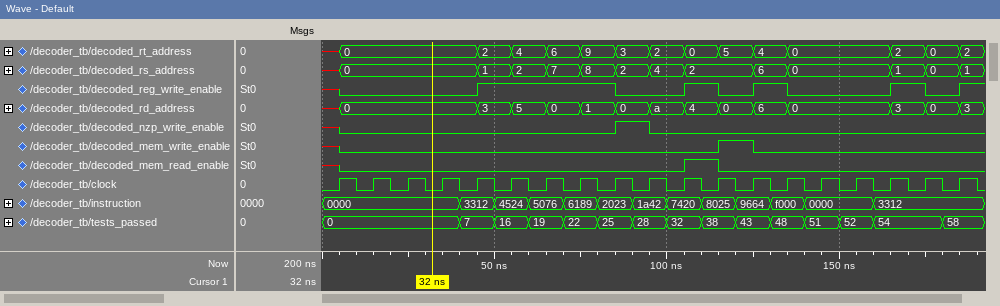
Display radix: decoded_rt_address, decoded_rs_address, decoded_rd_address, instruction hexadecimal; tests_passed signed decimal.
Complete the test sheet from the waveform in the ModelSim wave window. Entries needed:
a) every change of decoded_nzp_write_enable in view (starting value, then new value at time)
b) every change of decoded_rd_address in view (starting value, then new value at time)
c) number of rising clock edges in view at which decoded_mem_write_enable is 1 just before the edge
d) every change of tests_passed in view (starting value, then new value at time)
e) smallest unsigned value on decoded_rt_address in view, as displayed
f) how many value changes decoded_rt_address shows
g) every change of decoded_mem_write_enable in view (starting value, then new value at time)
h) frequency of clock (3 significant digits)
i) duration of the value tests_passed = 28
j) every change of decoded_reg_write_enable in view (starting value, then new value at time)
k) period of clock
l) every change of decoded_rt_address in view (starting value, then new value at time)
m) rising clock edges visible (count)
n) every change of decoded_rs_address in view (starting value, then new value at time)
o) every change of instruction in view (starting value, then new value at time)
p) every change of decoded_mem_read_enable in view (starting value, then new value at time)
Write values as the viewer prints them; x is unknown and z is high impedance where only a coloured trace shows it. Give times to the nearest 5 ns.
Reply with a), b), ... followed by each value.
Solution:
a) x, 0 at 5 ns, 1 at 85 ns, 0 at 95 ns
b) x, 0 at 5 ns, 3 at 45 ns, 5 at 55 ns, 0 at 65 ns, 1 at 75 ns, 0 at 85 ns, a at 95 ns, 4 at 105 ns, 0 at 115 ns, 6 at 125 ns, 0 at 135 ns, 3 at 165 ns, 0 at 175 ns, 3 at 185 ns
c) 1
d) 0, 7 at 40 ns, 16 at 50 ns, 19 at 60 ns, 22 at 70 ns, 25 at 80 ns, 28 at 90 ns, 32 at 100 ns, 38 at 110 ns, 43 at 120 ns, 48 at 130 ns, 51 at 140 ns, 52 at 150 ns, 54 at 160 ns, 58 at 180 ns
e) 0
f) 14
g) x, 0 at 5 ns, 1 at 115 ns, 0 at 125 ns
h) 100 MHz
i) 10 ns
j) x, 0 at 5 ns, 1 at 45 ns, 0 at 85 ns, 1 at 105 ns, 0 at 115 ns, 1 at 125 ns, 0 at 135 ns, 1 at 165 ns, 0 at 175 ns, 1 at 185 ns
k) 10 ns
l) x, 0 at 5 ns, 2 at 45 ns, 4 at 55 ns, 6 at 65 ns, 9 at 75 ns, 3 at 85 ns, 2 at 95 ns, 0 at 105 ns, 5 at 115 ns, 4 at 125 ns, 0 at 135 ns, 2 at 165 ns, 0 at 175 ns, 2 at 185 ns
m) 19
n) x, 0 at 5 ns, 1 at 45 ns, 2 at 55 ns, 7 at 65 ns, 8 at 75 ns, 2 at 85 ns, 4 at 95 ns, 2 at 105 ns, 6 at 125 ns, 0 at 135 ns, 1 at 165 ns, 0 at 175 ns, 1 at 185 ns
o) 0000, 3312 at 40 ns, 4524 at 50 ns, 5076 at 60 ns, 6189 at 70 ns, 2023 at 80 ns, 1a42 at 90 ns, 7420 at 100 ns, 8025 at 110 ns, 9664 at 120 ns, f000 at 130 ns, 0000 at 140 ns, 3312 at 160 ns
p) x, 0 at 5 ns, 1 at 105 ns, 0 at 115 ns
